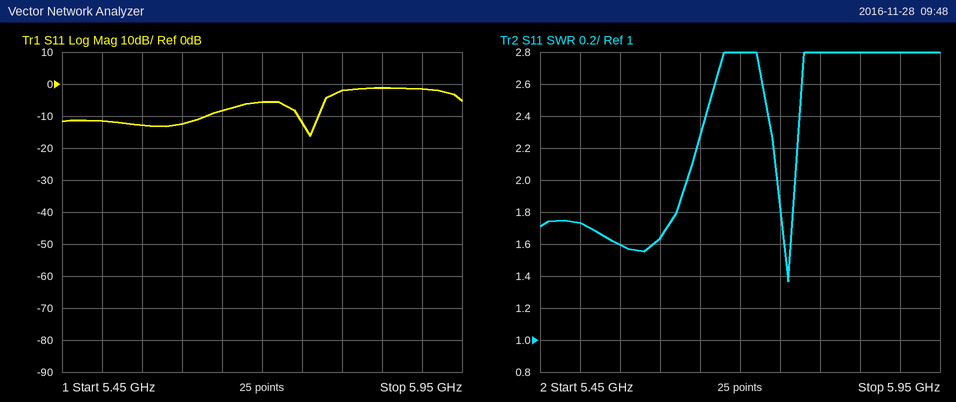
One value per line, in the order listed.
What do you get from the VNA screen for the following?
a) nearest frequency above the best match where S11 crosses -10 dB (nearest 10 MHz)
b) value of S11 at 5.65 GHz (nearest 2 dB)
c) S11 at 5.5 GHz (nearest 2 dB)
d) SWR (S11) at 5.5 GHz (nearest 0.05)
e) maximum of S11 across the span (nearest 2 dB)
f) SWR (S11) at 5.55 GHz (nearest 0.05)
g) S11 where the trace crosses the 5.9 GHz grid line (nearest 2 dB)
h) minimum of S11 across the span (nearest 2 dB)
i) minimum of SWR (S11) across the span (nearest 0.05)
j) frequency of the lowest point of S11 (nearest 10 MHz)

5.77 GHz
-8 dB
-12 dB
1.75
-2 dB
1.60
-2 dB
-16 dB
1.35
5.76 GHz
